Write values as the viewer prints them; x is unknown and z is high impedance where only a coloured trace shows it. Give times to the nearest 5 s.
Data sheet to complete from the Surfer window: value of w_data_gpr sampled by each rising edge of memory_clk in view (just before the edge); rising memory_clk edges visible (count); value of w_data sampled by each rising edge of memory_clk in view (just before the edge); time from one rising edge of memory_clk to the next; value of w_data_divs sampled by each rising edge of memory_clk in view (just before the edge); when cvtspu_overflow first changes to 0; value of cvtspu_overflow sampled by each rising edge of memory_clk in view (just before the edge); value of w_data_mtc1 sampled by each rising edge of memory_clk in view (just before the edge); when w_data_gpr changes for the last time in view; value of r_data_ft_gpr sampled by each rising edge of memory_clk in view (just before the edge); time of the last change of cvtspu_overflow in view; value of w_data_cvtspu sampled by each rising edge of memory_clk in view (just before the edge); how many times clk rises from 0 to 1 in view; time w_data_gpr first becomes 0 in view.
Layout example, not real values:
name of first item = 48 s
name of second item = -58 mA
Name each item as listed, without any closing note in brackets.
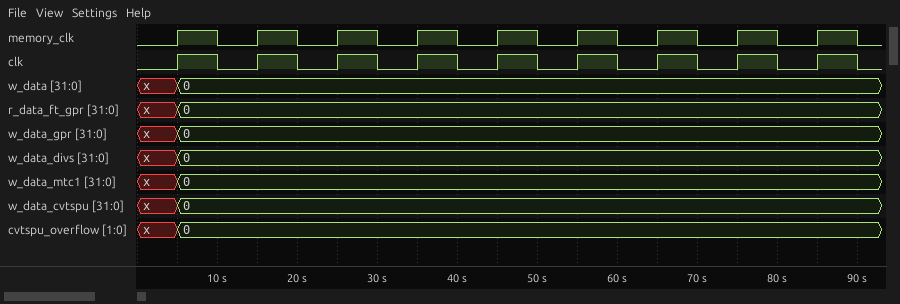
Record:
value of w_data_gpr sampled by each rising edge of memory_clk in view = x, 0, 0, 0, 0, 0, 0, 0, 0
rising memory_clk edges visible = 9
value of w_data sampled by each rising edge of memory_clk in view = x, 0, 0, 0, 0, 0, 0, 0, 0
time from one rising edge of memory_clk to the next = 10 s
value of w_data_divs sampled by each rising edge of memory_clk in view = x, 0, 0, 0, 0, 0, 0, 0, 0
when cvtspu_overflow first changes to 0 = 5 s
value of cvtspu_overflow sampled by each rising edge of memory_clk in view = x, 0, 0, 0, 0, 0, 0, 0, 0
value of w_data_mtc1 sampled by each rising edge of memory_clk in view = x, 0, 0, 0, 0, 0, 0, 0, 0
when w_data_gpr changes for the last time in view = 5 s
value of r_data_ft_gpr sampled by each rising edge of memory_clk in view = x, 0, 0, 0, 0, 0, 0, 0, 0
time of the last change of cvtspu_overflow in view = 5 s
value of w_data_cvtspu sampled by each rising edge of memory_clk in view = x, 0, 0, 0, 0, 0, 0, 0, 0
how many times clk rises from 0 to 1 in view = 9
time w_data_gpr first becomes 0 in view = 5 s
